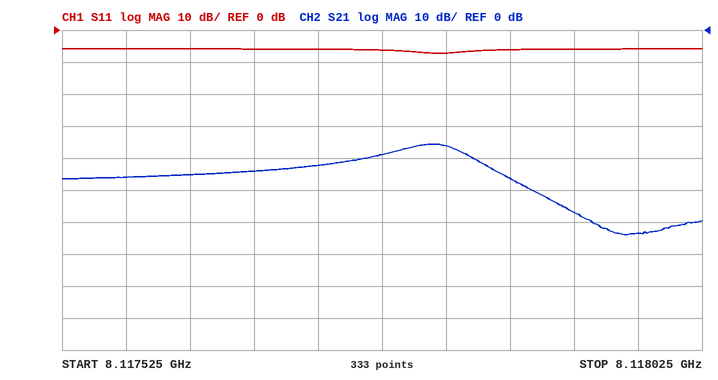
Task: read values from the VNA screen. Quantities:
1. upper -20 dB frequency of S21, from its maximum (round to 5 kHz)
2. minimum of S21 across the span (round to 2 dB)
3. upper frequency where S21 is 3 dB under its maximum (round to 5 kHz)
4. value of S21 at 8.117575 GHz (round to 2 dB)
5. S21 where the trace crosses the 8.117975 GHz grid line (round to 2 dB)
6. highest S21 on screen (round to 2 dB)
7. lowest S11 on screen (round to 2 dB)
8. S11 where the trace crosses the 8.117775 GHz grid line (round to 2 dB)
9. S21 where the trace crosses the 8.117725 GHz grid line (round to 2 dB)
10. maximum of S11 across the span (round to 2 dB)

8.117920 GHz
-64 dB
8.117840 GHz
-46 dB
-64 dB
-36 dB
-8 dB
-6 dB
-42 dB
-6 dB
